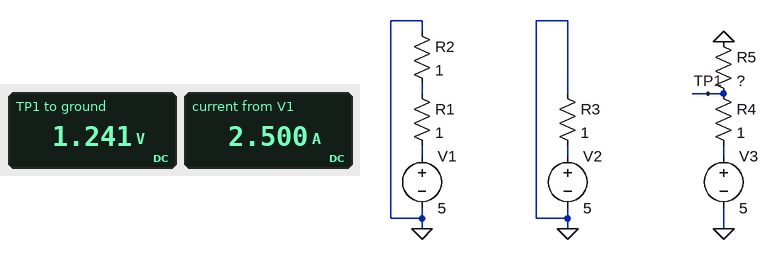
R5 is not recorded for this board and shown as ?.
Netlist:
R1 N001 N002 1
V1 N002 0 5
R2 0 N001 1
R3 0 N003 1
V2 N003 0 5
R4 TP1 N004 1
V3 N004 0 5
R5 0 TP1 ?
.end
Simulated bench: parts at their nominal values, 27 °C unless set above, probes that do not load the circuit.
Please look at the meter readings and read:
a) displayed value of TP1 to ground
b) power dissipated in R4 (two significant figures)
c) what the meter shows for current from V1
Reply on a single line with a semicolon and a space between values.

1.241 V; 14 W; 2.500 A
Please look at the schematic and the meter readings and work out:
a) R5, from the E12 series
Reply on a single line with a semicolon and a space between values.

0.33 Ω
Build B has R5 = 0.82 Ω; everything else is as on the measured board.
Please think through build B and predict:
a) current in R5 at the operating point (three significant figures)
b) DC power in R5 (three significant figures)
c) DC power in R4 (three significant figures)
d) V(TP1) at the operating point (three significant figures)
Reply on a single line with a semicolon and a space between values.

2.75 A; 6.19 W; 7.55 W; 2.25 V
